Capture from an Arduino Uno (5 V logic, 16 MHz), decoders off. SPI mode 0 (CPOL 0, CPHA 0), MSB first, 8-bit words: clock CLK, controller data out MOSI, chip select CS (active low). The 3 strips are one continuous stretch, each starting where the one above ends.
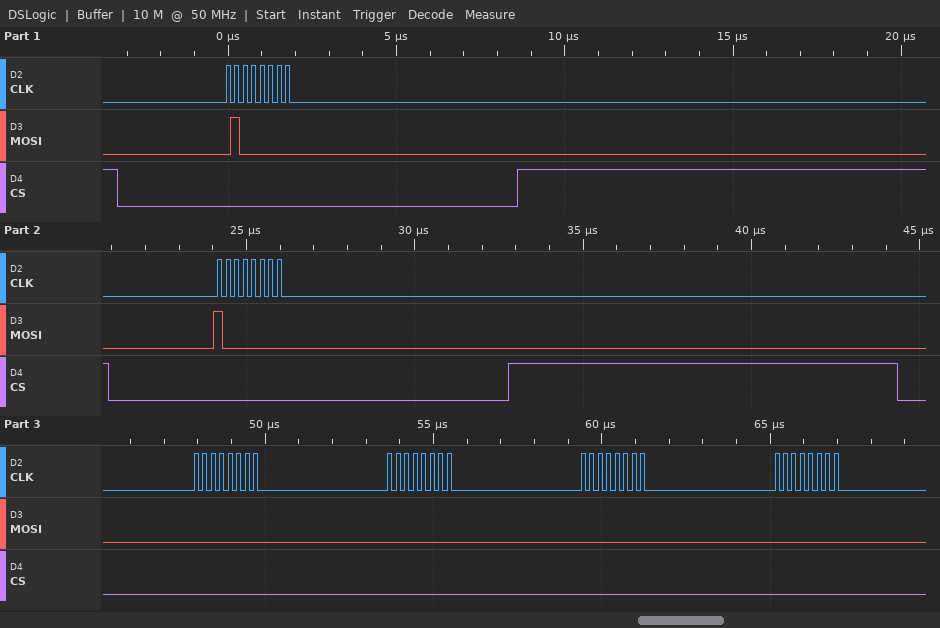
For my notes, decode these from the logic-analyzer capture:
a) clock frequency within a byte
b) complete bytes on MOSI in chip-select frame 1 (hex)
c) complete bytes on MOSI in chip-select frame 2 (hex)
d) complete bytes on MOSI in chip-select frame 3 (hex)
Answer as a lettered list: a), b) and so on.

a) 4 MHz
b) 0x40
c) 0x80
d) 0x00 0x00 0x00 0x00
